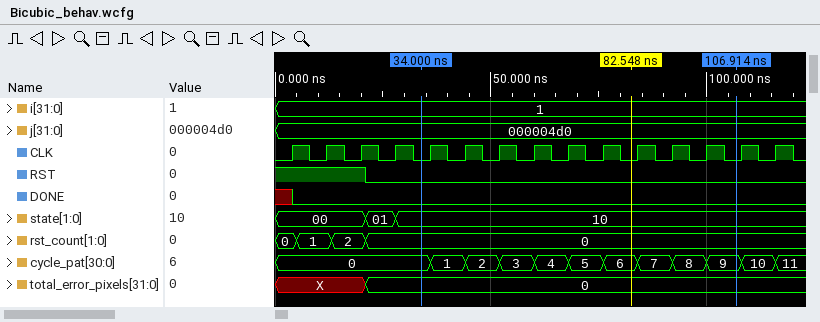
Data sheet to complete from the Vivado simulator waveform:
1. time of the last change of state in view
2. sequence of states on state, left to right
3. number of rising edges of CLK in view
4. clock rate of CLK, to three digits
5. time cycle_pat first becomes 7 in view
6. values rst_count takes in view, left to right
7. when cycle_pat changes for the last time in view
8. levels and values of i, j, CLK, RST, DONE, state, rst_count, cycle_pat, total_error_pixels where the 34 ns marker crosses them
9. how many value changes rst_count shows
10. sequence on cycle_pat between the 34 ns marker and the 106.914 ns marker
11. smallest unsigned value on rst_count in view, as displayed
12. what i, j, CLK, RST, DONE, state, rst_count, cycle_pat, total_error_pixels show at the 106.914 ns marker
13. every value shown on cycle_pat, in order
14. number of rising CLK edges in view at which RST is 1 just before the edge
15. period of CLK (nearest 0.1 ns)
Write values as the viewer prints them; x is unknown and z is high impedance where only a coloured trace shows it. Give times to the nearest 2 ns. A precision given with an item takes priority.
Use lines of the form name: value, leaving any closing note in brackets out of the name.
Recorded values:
time of the last change of state in view: 28 ns
sequence of states on state, left to right: 00, 01, 10
number of rising edges of CLK in view: 15
clock rate of CLK, to three digits: 125 MHz
time cycle_pat first becomes 7 in view: 84 ns
values rst_count takes in view, left to right: 0, 1, 2, 0
when cycle_pat changes for the last time in view: 116 ns
levels and values of i, j, CLK, RST, DONE, state, rst_count, cycle_pat, total_error_pixels where the 34 ns marker crosses them: i=1, j=000004d0, CLK=0, RST=0, DONE=0, state=10, rst_count=0, cycle_pat=0, total_error_pixels=0
how many value changes rst_count shows: 3
sequence on cycle_pat between the 34 ns marker and the 106.914 ns marker: 0, 1, 2, 3, 4, 5, 6, 7, 8, 9
smallest unsigned value on rst_count in view, as displayed: 0
what i, j, CLK, RST, DONE, state, rst_count, cycle_pat, total_error_pixels show at the 106.914 ns marker: i=1, j=000004d0, CLK=0, RST=0, DONE=0, state=10, rst_count=0, cycle_pat=9, total_error_pixels=0
every value shown on cycle_pat, in order: 0, 1, 2, 3, 4, 5, 6, 7, 8, 9, 10, 11
number of rising CLK edges in view at which RST is 1 just before the edge: 3
period of CLK: 8 ns
